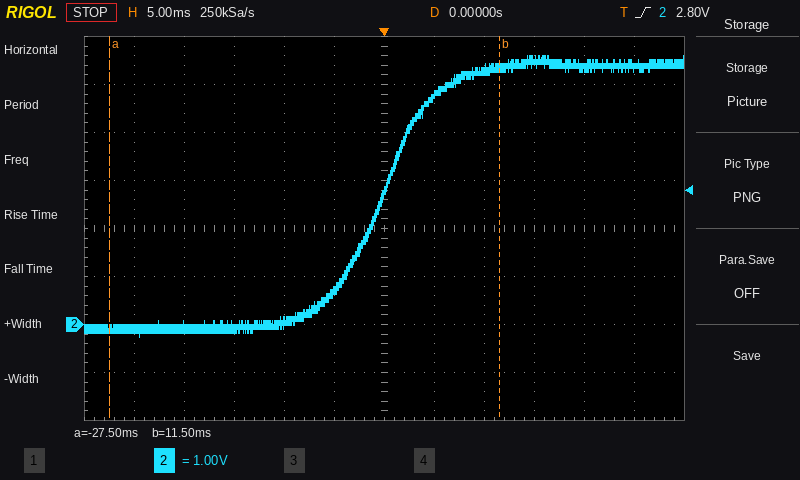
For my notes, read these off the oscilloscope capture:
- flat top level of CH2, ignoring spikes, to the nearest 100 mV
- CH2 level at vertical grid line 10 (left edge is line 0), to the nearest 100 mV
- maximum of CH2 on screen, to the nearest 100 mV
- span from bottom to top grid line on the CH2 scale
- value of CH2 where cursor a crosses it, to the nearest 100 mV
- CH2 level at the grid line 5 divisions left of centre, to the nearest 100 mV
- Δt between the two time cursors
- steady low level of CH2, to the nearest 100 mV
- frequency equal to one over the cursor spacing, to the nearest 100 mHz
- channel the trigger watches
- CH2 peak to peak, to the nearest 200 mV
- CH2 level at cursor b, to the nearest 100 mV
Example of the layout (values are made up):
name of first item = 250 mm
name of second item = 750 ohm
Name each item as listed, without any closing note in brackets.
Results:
flat top level of CH2, ignoring spikes, to the nearest 100 mV = 5.4 V
CH2 level at vertical grid line 10 (left edge is line 0), to the nearest 100 mV = 5.4 V
maximum of CH2 on screen, to the nearest 100 mV = 5.6 V
span from bottom to top grid line on the CH2 scale = 8 V
value of CH2 where cursor a crosses it, to the nearest 100 mV = -100 mV
CH2 level at the grid line 5 divisions left of centre, to the nearest 100 mV = -100 mV
Δt between the two time cursors = 39.0 ms
steady low level of CH2, to the nearest 100 mV = -100 mV
frequency equal to one over the cursor spacing, to the nearest 100 mHz = 25.6 Hz
channel the trigger watches = CH2
CH2 peak to peak, to the nearest 200 mV = 5.8 V
CH2 level at cursor b, to the nearest 100 mV = 5.4 V
